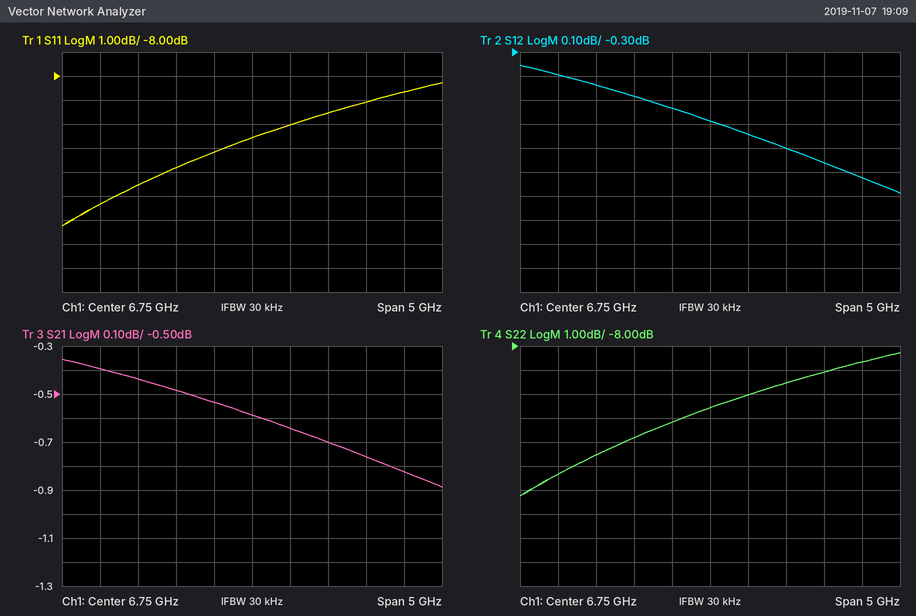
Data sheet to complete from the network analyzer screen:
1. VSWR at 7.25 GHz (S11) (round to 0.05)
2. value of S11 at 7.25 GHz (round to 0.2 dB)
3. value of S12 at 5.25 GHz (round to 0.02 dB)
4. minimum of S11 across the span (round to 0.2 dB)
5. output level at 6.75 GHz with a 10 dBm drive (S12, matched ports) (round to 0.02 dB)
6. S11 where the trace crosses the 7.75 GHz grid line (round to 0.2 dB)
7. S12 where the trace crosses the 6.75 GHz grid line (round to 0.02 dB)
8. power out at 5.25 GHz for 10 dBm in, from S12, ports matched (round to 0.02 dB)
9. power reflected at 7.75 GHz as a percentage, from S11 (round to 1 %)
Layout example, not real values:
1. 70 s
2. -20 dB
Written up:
1. 1.90
2. -10.0 dB
3. -0.44 dB
4. -14.2 dB
5. 9.42 dBm
6. -9.6 dB
7. -0.58 dB
8. 9.56 dBm
9. 11 %
